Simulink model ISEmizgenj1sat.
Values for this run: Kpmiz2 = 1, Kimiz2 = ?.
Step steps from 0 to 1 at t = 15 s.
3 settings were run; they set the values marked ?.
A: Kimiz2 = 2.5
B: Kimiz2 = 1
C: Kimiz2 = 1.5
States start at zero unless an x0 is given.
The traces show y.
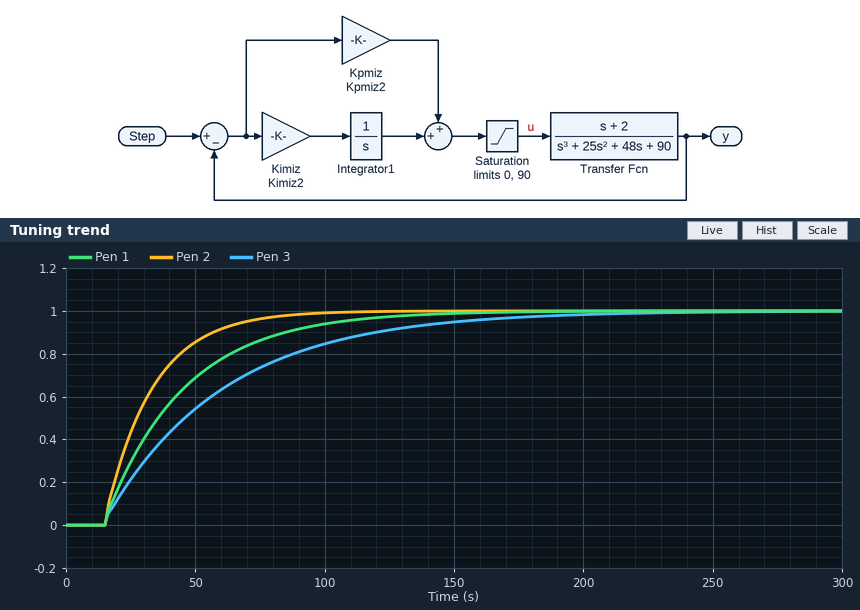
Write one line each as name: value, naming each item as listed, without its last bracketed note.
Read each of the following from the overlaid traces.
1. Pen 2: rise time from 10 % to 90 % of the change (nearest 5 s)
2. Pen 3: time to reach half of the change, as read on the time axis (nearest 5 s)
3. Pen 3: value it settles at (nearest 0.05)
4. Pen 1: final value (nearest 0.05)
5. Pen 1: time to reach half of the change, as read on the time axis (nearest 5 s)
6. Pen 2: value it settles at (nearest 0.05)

Pen 2: rise time from 10 % to 90 % of the change: 40 s
Pen 3: time to reach half of the change, as read on the time axis: 45 s
Pen 3: value it settles at: 1.00
Pen 1: final value: 1.00
Pen 1: time to reach half of the change, as read on the time axis: 35 s
Pen 2: value it settles at: 1.00
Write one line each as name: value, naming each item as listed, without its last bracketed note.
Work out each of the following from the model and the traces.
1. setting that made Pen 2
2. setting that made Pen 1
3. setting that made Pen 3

setting that made Pen 2: A
setting that made Pen 1: C
setting that made Pen 3: B
